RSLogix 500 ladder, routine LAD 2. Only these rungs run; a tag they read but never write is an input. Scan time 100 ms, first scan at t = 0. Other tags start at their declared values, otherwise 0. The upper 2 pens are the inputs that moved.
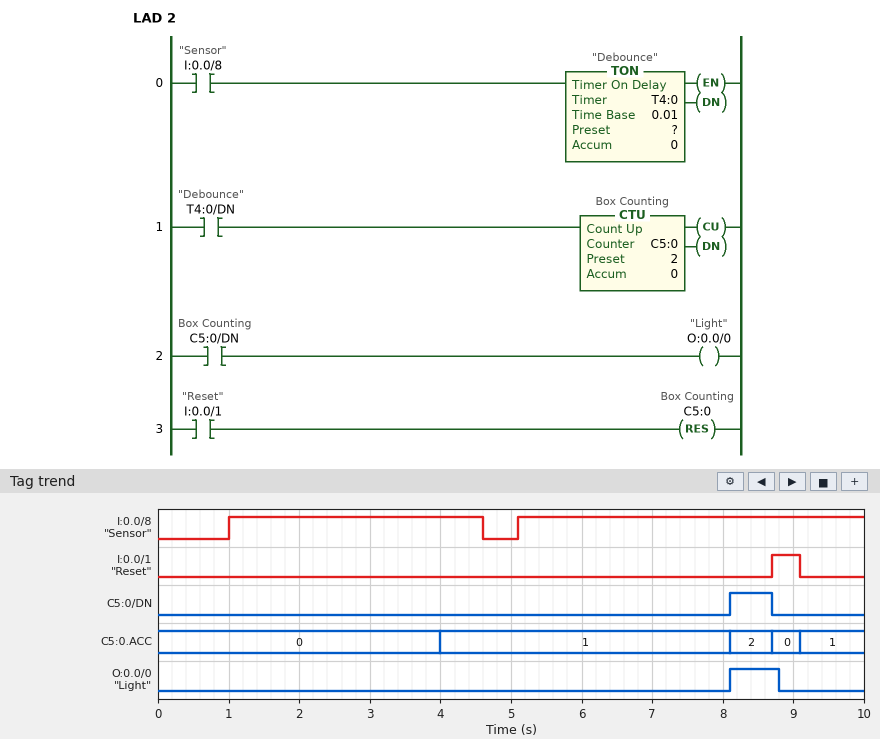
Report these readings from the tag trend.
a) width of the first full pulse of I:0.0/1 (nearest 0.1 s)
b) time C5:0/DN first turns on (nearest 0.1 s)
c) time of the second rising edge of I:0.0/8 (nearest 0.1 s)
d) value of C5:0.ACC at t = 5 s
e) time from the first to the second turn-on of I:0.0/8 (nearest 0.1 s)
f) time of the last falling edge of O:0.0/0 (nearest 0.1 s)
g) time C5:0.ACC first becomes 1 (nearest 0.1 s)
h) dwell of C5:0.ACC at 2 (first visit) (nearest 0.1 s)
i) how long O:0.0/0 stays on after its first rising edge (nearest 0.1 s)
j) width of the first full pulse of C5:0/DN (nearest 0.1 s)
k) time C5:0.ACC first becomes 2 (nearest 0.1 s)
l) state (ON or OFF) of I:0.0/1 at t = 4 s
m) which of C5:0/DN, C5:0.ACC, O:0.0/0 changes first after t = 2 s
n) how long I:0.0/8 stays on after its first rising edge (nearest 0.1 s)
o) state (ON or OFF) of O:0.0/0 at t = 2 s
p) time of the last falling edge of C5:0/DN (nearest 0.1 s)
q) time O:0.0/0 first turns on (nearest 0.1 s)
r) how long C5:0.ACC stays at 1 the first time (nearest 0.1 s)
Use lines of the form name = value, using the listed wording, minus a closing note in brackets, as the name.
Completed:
width of the first full pulse of I:0.0/1 = 0.4 s
time C5:0/DN first turns on = 8.1 s
time of the second rising edge of I:0.0/8 = 5.1 s
value of C5:0.ACC at t = 5 s = 1
time from the first to the second turn-on of I:0.0/8 = 4.1 s
time of the last falling edge of O:0.0/0 = 8.8 s
time C5:0.ACC first becomes 1 = 4.0 s
dwell of C5:0.ACC at 2 (first visit) = 0.6 s
how long O:0.0/0 stays on after its first rising edge = 0.7 s
width of the first full pulse of C5:0/DN = 0.6 s
time C5:0.ACC first becomes 2 = 8.1 s
state (ON or OFF) of I:0.0/1 at t = 4 s = OFF
which of C5:0/DN, C5:0.ACC, O:0.0/0 changes first after t = 2 s = C5:0.ACC
how long I:0.0/8 stays on after its first rising edge = 3.6 s
state (ON or OFF) of O:0.0/0 at t = 2 s = OFF
time of the last falling edge of C5:0/DN = 8.7 s
time O:0.0/0 first turns on = 8.1 s
how long C5:0.ACC stays at 1 the first time = 4.1 s
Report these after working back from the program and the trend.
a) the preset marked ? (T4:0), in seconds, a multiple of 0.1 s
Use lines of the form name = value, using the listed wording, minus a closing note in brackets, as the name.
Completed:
the preset marked ? (T4:0), in seconds, a multiple of 0.1 s = 3.0 s
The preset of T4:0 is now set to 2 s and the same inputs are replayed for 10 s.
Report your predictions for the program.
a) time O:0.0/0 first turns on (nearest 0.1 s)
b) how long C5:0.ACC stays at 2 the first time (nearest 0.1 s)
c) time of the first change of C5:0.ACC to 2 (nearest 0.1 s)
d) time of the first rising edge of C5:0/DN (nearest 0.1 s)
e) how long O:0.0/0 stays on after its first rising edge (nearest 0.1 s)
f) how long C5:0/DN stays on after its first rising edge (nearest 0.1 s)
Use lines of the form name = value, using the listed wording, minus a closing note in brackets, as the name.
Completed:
time O:0.0/0 first turns on = 7.1 s
how long C5:0.ACC stays at 2 the first time = 1.6 s
time of the first change of C5:0.ACC to 2 = 7.1 s
time of the first rising edge of C5:0/DN = 7.1 s
how long O:0.0/0 stays on after its first rising edge = 1.7 s
how long C5:0/DN stays on after its first rising edge = 1.6 s
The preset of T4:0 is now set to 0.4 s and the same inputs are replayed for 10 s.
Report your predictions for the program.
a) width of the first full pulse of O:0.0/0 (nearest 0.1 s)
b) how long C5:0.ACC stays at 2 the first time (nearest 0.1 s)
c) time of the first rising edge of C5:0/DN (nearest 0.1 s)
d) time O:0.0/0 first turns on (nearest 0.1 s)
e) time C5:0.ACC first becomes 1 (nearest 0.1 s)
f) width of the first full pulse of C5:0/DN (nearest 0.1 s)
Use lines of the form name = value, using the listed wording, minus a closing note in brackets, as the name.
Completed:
width of the first full pulse of O:0.0/0 = 3.3 s
how long C5:0.ACC stays at 2 the first time = 3.2 s
time of the first rising edge of C5:0/DN = 5.5 s
time O:0.0/0 first turns on = 5.5 s
time C5:0.ACC first becomes 1 = 1.4 s
width of the first full pulse of C5:0/DN = 3.2 s
